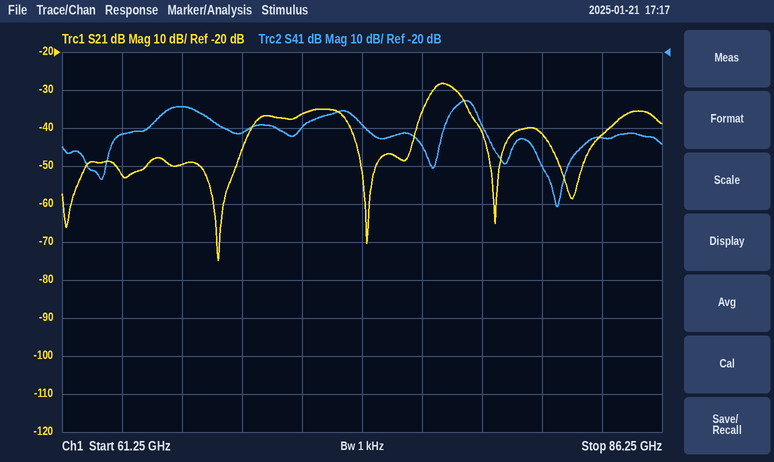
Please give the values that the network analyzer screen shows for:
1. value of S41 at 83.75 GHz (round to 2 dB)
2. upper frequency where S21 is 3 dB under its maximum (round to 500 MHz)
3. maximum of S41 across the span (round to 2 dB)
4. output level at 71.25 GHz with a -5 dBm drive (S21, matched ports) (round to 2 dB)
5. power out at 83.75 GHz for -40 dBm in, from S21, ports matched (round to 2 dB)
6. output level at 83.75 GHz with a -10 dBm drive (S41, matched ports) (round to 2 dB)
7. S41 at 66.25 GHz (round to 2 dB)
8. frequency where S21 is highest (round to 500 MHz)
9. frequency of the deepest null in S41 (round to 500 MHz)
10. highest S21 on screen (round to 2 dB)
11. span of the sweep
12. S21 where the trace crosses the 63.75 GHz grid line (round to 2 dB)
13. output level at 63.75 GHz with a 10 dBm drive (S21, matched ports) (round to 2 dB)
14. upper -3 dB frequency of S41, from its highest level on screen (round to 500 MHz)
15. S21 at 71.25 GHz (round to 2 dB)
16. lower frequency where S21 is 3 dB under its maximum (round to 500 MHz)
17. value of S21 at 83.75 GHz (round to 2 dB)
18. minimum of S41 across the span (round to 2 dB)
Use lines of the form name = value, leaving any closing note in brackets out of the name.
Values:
value of S41 at 83.75 GHz = -42 dB
upper frequency where S21 is 3 dB under its maximum = 78.0 GHz
maximum of S41 across the span = -32 dB
output level at 71.25 GHz with a -5 dBm drive (S21, matched ports) = -42 dBm
power out at 83.75 GHz for -40 dBm in, from S21, ports matched = -82 dBm
output level at 83.75 GHz with a -10 dBm drive (S41, matched ports) = -52 dBm
S41 at 66.25 GHz = -34 dB
frequency where S21 is highest = 77.0 GHz
frequency of the deepest null in S41 = 82.0 GHz
highest S21 on screen = -28 dB
span of the sweep = 25 GHz
S21 where the trace crosses the 63.75 GHz grid line = -52 dB
output level at 63.75 GHz with a 10 dBm drive (S21, matched ports) = -42 dBm
upper -3 dB frequency of S41, from its highest level on screen = 78.5 GHz
S21 at 71.25 GHz = -36 dB
lower frequency where S21 is 3 dB under its maximum = 76.5 GHz
value of S21 at 83.75 GHz = -42 dB
minimum of S41 across the span = -60 dB
